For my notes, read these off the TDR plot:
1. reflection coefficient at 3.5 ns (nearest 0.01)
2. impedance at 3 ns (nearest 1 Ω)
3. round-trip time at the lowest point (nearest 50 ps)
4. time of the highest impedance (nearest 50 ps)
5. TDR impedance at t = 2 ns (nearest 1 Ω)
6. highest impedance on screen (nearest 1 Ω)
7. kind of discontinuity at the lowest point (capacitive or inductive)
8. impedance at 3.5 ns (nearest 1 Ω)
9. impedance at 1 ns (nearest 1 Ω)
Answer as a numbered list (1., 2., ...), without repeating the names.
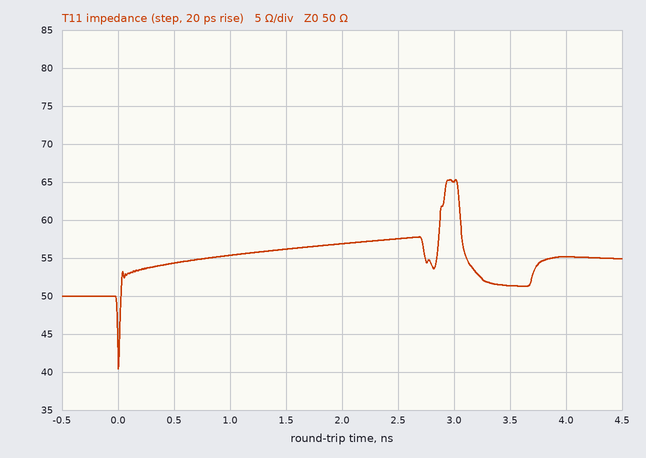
1. +0.01
2. 65 Ω
3. 0 ps
4. 3.00 ns
5. 57 Ω
6. 65 Ω
7. capacitive
8. 51 Ω
9. 55 Ω
